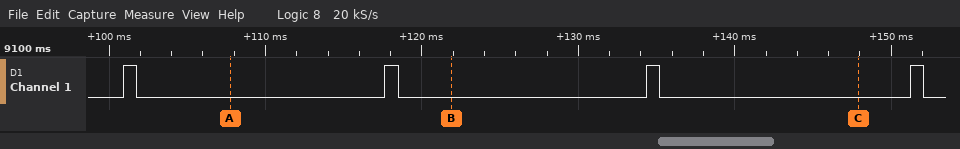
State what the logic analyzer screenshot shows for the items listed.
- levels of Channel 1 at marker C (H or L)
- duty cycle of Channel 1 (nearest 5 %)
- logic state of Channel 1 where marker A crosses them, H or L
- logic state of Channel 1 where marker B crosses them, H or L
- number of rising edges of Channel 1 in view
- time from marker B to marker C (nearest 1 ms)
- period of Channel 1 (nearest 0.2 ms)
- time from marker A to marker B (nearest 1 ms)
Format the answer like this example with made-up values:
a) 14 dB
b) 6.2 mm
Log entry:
a) Channel 1=L
b) 5 %
c) Channel 1=L
d) Channel 1=L
e) 4
f) 26 ms
g) 16.8 ms
h) 14 ms
